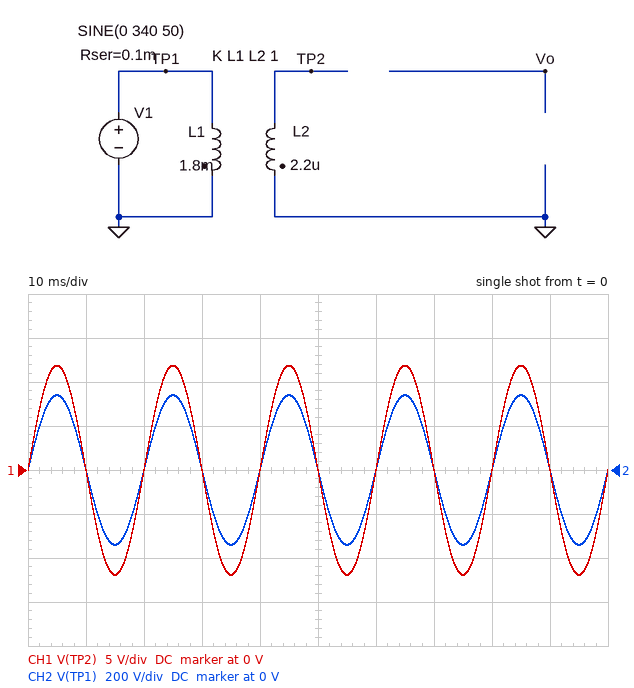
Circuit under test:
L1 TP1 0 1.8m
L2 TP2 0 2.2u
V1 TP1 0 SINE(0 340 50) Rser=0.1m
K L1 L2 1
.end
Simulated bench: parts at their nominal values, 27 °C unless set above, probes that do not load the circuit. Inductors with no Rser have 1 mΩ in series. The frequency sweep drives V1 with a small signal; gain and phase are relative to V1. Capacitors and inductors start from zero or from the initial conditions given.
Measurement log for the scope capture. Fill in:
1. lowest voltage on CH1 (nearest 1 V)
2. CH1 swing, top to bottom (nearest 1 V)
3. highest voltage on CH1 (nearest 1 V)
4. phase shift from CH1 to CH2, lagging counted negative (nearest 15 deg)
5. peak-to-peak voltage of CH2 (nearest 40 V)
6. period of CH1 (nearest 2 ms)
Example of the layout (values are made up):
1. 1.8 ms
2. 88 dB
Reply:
1. -12 V
2. 24 V
3. 12 V
4. 0 deg
5. 680 V
6. 20 ms
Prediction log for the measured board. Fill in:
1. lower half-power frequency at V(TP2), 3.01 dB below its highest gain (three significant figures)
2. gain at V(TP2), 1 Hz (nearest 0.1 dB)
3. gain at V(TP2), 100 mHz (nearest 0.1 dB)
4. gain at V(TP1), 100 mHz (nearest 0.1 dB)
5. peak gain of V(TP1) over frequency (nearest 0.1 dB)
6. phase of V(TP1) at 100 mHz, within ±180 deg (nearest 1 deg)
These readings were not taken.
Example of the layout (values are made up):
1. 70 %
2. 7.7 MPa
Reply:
1. 97.3 mHz
2. -29.2 dB
3. -32.0 dB
4. -0.4 dB
5. 0 dB
6. 3 deg
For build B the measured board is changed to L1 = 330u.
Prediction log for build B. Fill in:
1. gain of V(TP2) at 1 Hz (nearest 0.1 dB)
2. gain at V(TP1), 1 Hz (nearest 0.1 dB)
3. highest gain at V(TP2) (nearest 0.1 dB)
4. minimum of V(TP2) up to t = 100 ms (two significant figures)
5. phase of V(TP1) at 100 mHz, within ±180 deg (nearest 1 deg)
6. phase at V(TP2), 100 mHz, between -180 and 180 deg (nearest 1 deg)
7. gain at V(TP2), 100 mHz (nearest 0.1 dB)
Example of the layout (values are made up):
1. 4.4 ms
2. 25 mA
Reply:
1. -22.8 dB
2. -0.2 dB
3. -21.8 dB
4. -28 V
5. 1 deg
6. 79 deg
7. -36.4 dB
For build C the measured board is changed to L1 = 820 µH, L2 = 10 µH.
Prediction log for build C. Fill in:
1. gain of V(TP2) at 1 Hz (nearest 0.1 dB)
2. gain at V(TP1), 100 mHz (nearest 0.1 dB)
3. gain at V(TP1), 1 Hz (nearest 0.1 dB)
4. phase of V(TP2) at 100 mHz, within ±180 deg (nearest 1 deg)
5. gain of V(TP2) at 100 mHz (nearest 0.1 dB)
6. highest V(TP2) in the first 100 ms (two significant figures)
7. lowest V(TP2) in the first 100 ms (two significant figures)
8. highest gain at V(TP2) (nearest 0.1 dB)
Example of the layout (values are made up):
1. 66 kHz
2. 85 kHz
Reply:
1. -19.3 dB
2. -0.7 dB
3. 0 dB
4. 65 deg
5. -26.6 dB
6. 37 V
7. -38 V
8. -19.1 dB
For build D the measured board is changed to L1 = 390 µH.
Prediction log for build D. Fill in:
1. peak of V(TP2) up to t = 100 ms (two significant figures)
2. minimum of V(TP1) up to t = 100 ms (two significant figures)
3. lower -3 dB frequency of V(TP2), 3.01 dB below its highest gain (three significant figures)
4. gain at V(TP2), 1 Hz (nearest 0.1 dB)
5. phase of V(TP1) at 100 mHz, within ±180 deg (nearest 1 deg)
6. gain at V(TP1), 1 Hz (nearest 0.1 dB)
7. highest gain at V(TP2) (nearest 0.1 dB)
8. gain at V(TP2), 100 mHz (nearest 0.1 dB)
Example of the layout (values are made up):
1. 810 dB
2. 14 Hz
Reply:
1. 25 V
2. -340 V
3. 449 mHz
4. -23.3 dB
5. 1 deg
6. -0.1 dB
7. -22.5 dB
8. -35.7 dB
